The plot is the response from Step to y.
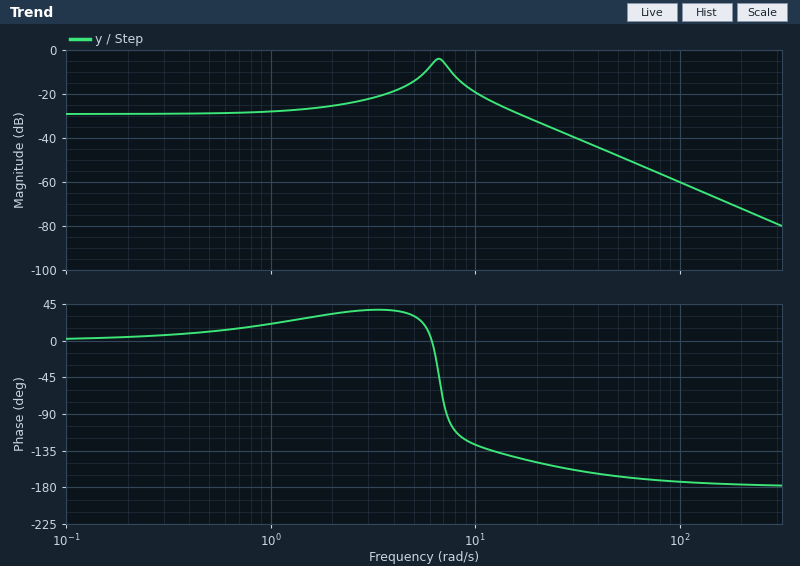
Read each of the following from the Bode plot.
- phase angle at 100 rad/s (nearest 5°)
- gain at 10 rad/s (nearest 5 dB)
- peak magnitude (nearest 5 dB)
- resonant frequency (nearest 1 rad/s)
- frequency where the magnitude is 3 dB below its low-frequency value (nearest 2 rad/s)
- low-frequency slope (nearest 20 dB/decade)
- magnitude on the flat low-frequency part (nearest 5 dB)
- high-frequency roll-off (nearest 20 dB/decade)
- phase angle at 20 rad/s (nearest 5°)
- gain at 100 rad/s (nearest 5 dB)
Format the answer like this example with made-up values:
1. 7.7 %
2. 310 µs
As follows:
1. -175°
2. -20 dB
3. -5 dB
4. 7 rad/s
5. 20 rad/s
6. 0 dB/decade
7. -30 dB
8. -40 dB/decade
9. -150°
10. -60 dB
